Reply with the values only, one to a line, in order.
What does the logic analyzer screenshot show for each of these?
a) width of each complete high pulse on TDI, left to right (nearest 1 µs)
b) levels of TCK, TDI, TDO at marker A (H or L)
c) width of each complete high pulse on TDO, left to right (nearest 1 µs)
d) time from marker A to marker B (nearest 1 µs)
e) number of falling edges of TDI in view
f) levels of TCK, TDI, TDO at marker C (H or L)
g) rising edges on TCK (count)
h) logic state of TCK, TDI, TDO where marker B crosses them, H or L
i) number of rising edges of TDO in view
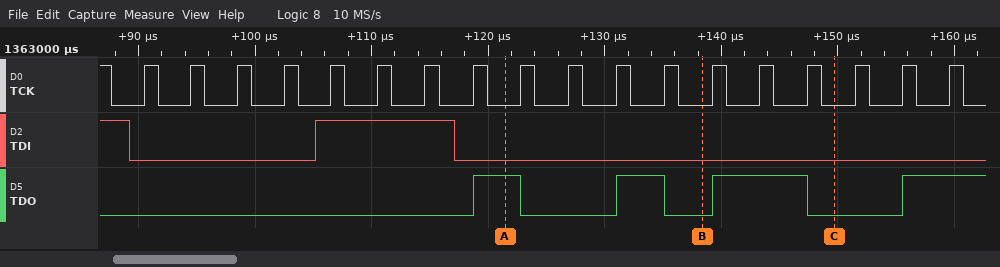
12 µs
TCK=L, TDI=L, TDO=H
4 µs, 4 µs, 8 µs
17 µs
2
TCK=L, TDI=L, TDO=L
18
TCK=L, TDI=L, TDO=L
4
